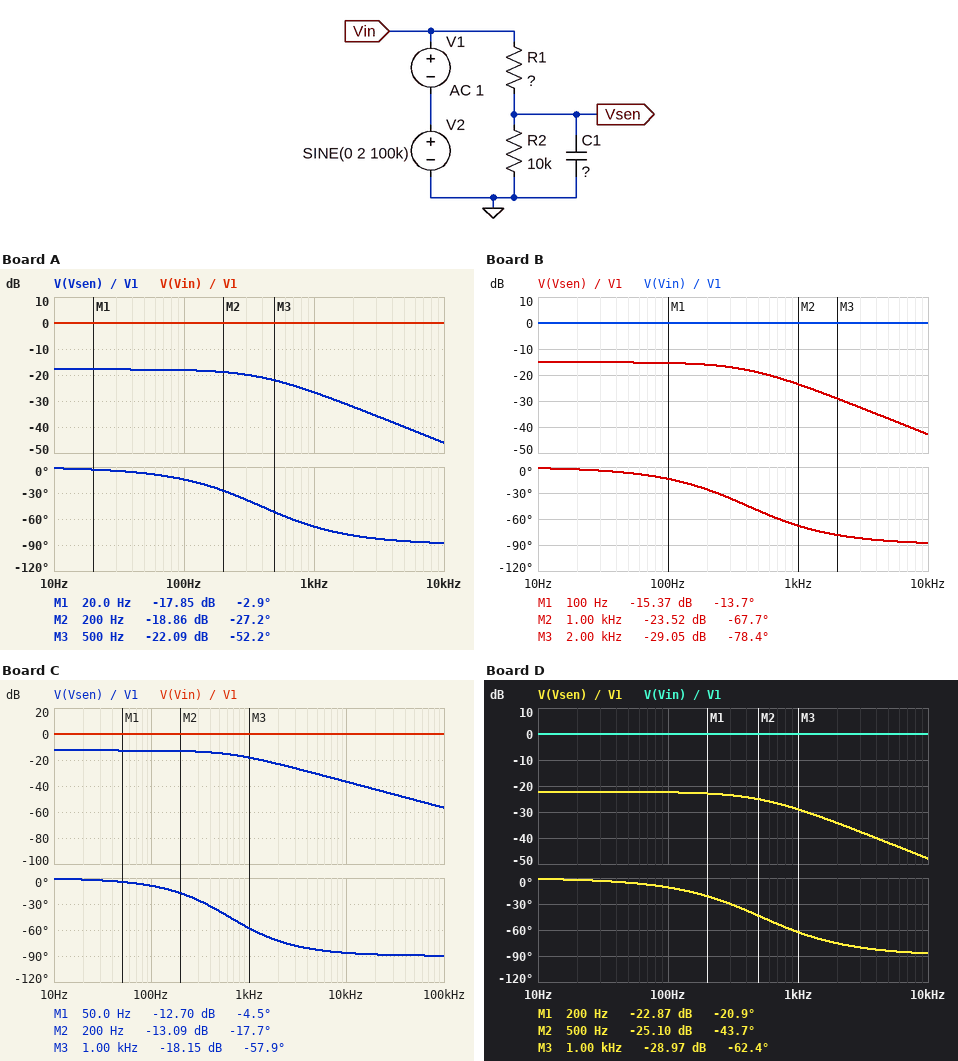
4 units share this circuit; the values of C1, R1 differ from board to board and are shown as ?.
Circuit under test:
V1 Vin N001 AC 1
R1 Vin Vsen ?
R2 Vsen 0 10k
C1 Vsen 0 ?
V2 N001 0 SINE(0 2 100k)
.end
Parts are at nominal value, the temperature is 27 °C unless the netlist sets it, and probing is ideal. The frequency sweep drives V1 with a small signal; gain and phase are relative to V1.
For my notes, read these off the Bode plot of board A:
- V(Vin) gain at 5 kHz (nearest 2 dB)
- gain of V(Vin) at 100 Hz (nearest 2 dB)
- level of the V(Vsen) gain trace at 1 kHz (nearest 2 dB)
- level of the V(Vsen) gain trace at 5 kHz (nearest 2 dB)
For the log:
0 dB
0 dB
-26 dB
-40 dB
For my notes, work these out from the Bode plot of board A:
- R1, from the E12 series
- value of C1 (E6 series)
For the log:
68 kΩ
47 nF
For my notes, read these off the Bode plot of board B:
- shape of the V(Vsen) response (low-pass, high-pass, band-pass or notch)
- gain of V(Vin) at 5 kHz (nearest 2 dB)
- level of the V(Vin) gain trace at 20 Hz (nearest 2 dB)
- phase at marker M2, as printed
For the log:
low-pass
0 dB
0 dB
-67.7 deg
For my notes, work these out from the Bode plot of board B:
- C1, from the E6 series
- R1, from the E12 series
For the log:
47 nF
47 kΩ
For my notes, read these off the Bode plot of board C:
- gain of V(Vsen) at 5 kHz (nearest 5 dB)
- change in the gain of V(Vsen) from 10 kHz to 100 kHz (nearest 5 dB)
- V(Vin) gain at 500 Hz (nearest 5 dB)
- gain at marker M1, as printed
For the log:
-30 dB
-20 dB
0 dB
-12.70 dB
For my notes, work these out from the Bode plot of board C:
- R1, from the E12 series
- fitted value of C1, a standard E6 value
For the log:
33 kΩ
33 nF
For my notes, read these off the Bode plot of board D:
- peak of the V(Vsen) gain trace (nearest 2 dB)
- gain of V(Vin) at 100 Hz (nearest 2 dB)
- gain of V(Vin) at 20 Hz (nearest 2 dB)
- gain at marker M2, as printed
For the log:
-22 dB
0 dB
0 dB
-25.10 dB
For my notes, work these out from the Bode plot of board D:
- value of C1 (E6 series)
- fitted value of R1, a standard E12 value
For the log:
33 nF
120 kΩ
